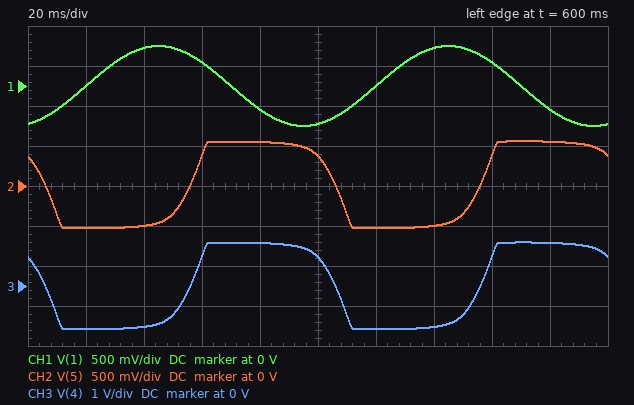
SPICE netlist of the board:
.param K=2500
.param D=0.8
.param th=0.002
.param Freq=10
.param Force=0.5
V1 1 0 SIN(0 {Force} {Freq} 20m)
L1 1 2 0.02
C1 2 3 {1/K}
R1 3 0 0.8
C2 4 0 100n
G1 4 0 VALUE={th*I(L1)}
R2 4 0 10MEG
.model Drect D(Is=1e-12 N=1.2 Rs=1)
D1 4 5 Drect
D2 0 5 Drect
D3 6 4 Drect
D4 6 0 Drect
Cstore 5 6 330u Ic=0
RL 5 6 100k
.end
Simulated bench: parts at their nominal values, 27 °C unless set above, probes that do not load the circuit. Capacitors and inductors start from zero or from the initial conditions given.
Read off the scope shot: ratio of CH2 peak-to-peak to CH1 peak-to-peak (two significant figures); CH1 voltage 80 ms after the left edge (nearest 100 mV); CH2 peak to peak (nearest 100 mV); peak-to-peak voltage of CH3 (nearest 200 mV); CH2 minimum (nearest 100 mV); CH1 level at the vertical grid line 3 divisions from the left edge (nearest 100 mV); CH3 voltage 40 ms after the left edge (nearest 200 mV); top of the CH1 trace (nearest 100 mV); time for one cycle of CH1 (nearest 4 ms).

1.1
-300 mV
1.1 V
2.2 V
-500 mV
300 mV
-1.0 V
500 mV
100 ms
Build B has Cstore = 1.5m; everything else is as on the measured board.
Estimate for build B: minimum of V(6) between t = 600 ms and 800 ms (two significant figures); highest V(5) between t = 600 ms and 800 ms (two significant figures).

-540 mV
540 mV
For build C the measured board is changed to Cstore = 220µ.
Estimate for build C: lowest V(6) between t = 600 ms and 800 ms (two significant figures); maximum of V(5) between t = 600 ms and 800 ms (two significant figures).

-570 mV
570 mV
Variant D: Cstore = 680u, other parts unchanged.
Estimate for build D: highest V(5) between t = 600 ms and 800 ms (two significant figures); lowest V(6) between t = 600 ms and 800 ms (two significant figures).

540 mV
-540 mV
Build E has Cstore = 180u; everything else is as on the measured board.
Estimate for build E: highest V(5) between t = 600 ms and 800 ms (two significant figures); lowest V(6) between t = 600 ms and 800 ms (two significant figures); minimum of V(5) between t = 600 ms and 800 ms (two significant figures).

580 mV
-580 mV
-530 mV
